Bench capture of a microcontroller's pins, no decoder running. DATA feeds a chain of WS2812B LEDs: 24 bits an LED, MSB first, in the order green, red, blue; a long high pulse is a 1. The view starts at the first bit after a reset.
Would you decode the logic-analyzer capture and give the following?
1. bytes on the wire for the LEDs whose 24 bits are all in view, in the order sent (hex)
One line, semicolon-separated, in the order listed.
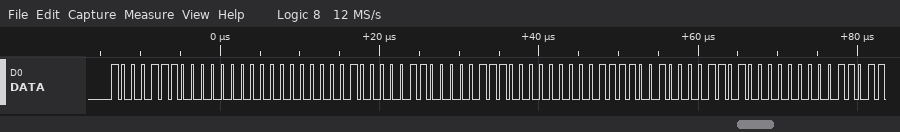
8E 00 00 83 07 00 79 0D 00
